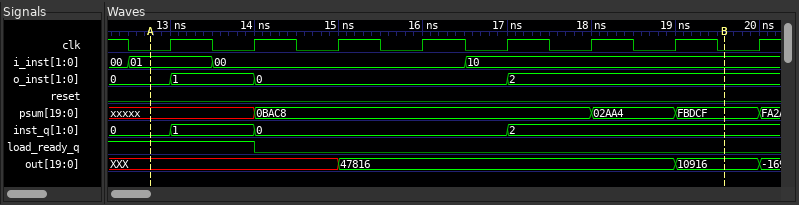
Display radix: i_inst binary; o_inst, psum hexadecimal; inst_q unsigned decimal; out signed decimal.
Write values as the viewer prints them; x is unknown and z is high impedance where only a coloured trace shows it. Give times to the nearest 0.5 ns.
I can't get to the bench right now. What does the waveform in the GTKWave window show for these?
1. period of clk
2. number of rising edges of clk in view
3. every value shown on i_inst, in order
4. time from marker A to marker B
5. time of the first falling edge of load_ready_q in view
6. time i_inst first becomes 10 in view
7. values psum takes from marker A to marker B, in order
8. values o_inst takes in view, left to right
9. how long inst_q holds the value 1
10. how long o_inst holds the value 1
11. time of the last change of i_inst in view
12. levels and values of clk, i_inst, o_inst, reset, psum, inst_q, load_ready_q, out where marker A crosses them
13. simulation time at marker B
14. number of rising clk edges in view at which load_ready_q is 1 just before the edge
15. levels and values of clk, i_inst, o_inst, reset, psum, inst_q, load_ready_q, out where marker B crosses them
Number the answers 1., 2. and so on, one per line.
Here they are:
1. 1 ns
2. 8
3. 00, 01, 00, 10
4. 7 ns
5. 14 ns
6. 16.5 ns
7. xxxxx, 0BAC8, 02AA4, FBDCF
8. 0, 1, 0, 2
9. 1 ns
10. 1 ns
11. 16.5 ns
12. clk=0, i_inst=01, o_inst=0, reset=0, psum=xxxxx, inst_q=0, load_ready_q=1, out=XXX
13. 19.5 ns
14. 2
15. clk=0, i_inst=10, o_inst=2, reset=0, psum=FBDCF, inst_q=2, load_ready_q=0, out=10916
